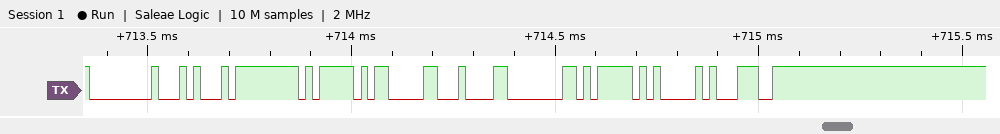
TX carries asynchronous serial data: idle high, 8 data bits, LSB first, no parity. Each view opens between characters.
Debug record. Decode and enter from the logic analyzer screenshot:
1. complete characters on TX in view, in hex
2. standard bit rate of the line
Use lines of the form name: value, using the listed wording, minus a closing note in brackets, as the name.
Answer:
complete characters on TX in view, in hex: 00, 14, FF, 7D, 83, 84, 80, 7D, 41, 9C
standard bit rate of the line: 57600 baud
